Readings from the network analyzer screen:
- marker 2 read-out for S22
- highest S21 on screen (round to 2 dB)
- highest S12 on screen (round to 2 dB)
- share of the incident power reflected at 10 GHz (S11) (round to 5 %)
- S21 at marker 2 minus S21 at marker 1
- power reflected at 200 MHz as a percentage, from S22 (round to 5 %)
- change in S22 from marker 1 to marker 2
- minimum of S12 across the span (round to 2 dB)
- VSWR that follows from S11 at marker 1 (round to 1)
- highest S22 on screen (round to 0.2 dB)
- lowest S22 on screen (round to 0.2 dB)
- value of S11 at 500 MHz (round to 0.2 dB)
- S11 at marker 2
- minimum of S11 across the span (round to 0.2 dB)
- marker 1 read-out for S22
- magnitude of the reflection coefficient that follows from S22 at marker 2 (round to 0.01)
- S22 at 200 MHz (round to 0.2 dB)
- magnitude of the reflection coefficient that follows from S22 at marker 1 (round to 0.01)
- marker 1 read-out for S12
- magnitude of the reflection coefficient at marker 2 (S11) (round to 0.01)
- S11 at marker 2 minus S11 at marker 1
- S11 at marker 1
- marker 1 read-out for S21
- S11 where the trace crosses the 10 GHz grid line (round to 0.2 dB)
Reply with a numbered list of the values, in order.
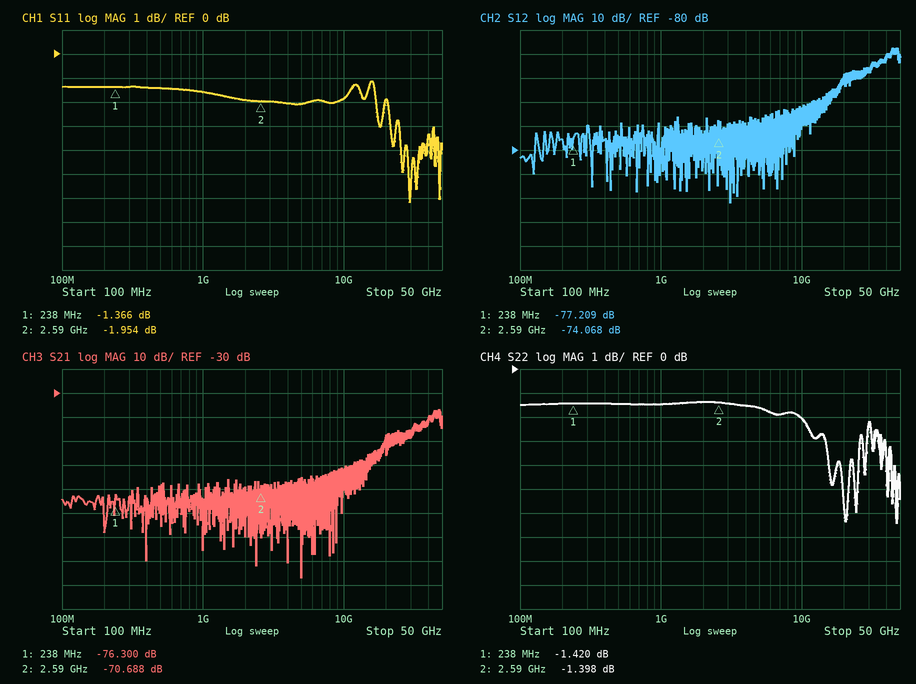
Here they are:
1. -1.398 dB
2. -36 dB
3. -38 dB
4. 65 %
5. 5.612 dB
6. 70 %
7. 0.022 dB
8. -102 dB
9. 13
10. -1.4 dB
11. -6.4 dB
12. -1.4 dB
13. -1.954 dB
14. -6.2 dB
15. -1.420 dB
16. 0.85
17. -1.4 dB
18. 0.85
19. -77.209 dB
20. 0.80
21. -0.588 dB
22. -1.366 dB
23. -76.300 dB
24. -1.8 dB
